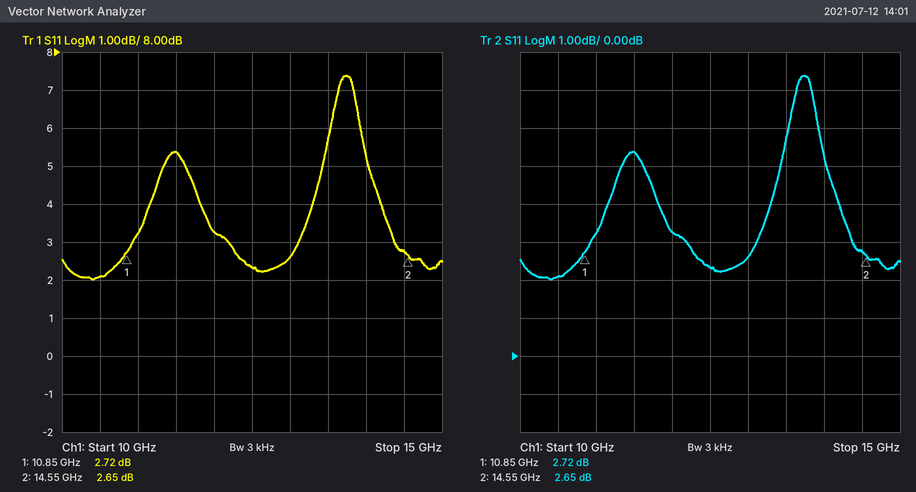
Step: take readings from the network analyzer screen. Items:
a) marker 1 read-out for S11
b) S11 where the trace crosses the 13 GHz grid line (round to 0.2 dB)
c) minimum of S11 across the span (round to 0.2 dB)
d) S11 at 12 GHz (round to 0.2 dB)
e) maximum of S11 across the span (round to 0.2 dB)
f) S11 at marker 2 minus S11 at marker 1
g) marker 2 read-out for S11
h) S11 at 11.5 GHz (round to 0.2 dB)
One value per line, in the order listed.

2.72 dB
2.6 dB
2.0 dB
3.2 dB
7.4 dB
-0.07 dB
2.65 dB
5.4 dB
